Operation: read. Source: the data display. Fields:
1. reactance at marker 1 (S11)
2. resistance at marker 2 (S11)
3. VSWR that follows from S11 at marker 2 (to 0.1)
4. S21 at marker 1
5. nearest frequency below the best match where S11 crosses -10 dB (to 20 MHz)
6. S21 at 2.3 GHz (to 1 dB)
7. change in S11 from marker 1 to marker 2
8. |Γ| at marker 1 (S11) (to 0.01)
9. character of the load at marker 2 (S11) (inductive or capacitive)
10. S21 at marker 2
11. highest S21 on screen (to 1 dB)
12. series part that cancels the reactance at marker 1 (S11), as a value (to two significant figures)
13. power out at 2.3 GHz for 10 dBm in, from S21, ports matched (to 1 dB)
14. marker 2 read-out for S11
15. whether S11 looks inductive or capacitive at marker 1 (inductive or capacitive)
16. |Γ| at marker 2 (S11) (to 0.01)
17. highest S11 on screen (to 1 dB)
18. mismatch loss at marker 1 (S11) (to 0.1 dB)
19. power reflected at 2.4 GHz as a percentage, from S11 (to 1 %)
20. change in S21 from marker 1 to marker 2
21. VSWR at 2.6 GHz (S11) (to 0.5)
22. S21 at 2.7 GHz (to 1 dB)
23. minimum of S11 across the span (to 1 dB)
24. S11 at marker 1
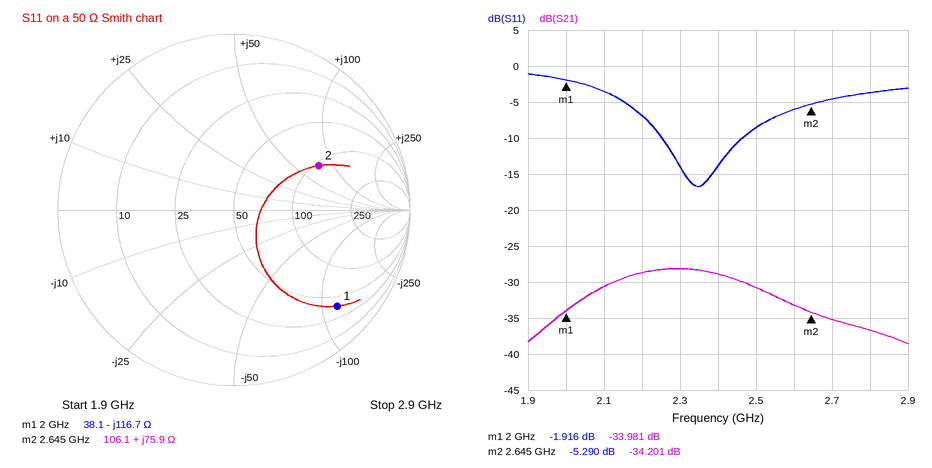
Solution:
-116.7 Ω
106.1 Ω
3.4
-33.981 dB
2.26 GHz
-28 dB
-3.374 dB
0.80
inductive
-34.201 dB
-28 dB
9.3 nH
-18 dBm
-5.290 dB
capacitive
0.54
-1 dB
4.5 dB
4 %
-0.220 dB
3.0
-35 dB
-17 dB
-1.916 dB
